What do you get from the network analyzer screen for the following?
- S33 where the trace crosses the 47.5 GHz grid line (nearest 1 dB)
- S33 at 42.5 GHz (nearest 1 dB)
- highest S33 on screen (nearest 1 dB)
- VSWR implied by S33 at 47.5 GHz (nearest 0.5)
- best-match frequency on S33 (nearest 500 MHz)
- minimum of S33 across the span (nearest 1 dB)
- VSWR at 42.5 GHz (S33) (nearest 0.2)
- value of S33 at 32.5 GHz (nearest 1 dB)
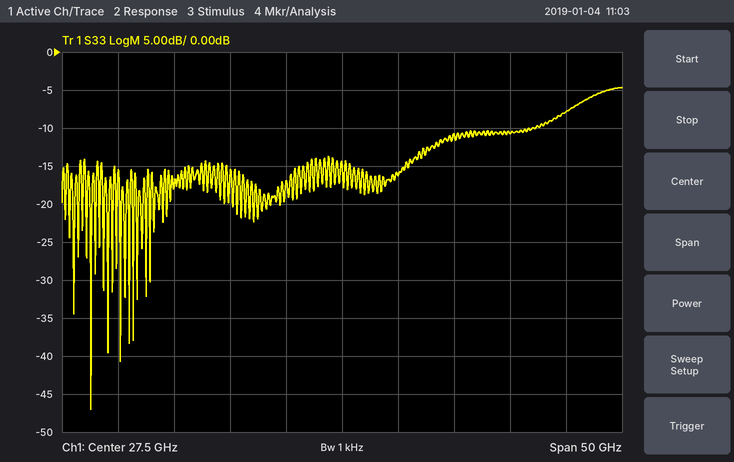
-8 dB
-11 dB
-5 dB
2.5
5.0 GHz
-47 dB
1.8
-16 dB
